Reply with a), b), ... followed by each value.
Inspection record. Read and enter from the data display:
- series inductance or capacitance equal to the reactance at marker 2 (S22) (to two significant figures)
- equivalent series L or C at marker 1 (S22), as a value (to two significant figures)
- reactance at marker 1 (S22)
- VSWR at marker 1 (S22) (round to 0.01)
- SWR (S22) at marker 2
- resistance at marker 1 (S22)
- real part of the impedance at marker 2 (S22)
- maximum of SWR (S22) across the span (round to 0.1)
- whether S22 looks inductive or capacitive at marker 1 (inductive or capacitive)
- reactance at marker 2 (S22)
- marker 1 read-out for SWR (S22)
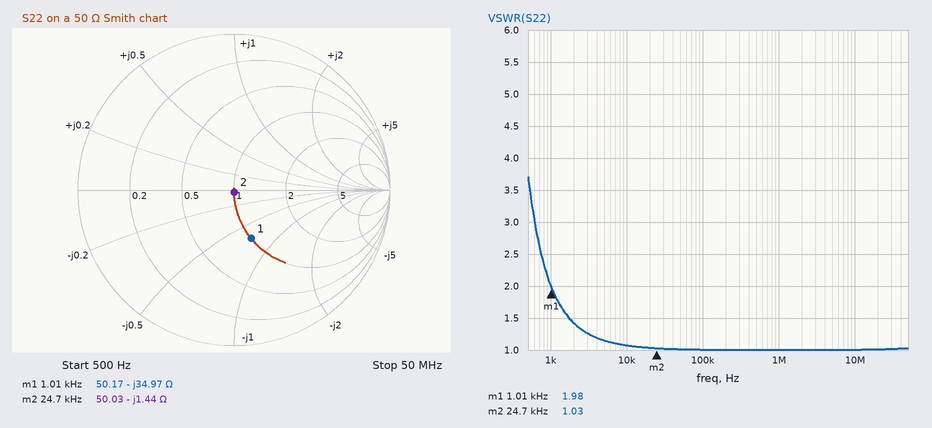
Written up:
a) 4.5 µF
b) 4.5 µF
c) -34.97 Ω
d) 1.98
e) 1.03
f) 50.17 Ω
g) 50.03 Ω
h) 3.7
i) capacitive
j) -1.44 Ω
k) 1.98
